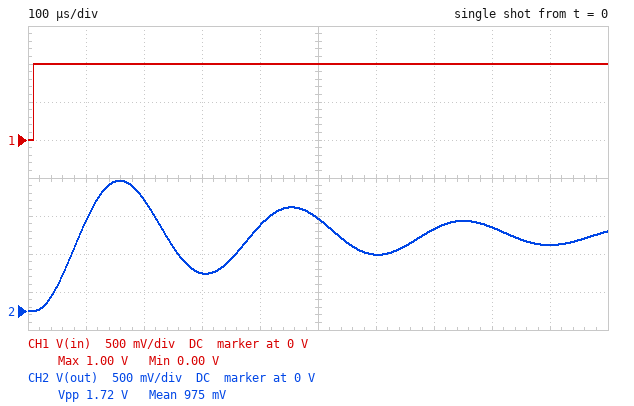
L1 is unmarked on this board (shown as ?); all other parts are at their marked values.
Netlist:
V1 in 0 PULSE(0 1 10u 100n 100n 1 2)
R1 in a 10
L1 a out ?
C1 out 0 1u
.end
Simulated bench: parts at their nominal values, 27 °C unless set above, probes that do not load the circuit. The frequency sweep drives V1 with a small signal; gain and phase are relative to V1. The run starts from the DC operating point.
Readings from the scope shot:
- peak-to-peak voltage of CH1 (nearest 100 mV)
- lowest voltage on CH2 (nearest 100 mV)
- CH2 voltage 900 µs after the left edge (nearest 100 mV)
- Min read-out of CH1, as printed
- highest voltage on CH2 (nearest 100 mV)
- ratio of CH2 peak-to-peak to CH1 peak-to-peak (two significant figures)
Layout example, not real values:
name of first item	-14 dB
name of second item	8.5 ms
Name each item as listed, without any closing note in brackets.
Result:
peak-to-peak voltage of CH1	1.0 V
lowest voltage on CH2	0 V
CH2 voltage 900 µs after the left edge	900 mV
Min read-out of CH1, as printed	0.00 V
highest voltage on CH2	1.7 V
ratio of CH2 peak-to-peak to CH1 peak-to-peak	1.7
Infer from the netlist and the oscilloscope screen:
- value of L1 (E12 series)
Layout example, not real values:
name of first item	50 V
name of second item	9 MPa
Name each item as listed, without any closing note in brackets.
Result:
value of L1	2.2 mH
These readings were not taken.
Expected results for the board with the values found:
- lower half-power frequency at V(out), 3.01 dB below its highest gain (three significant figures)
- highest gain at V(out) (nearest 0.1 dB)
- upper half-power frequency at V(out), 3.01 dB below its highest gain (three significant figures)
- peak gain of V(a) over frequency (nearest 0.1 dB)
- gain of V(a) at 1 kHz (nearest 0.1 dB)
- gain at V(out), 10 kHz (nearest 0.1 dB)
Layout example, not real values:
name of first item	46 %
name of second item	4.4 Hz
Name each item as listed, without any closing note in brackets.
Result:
lower half-power frequency at V(out), 3.01 dB below its highest gain	2.97 kHz
highest gain at V(out)	13.5 dB
upper half-power frequency at V(out), 3.01 dB below its highest gain	3.70 kHz
peak gain of V(a) over frequency	0 dB
gain of V(a) at 1 kHz	0 dB
gain at V(out), 10 kHz	-17.7 dB
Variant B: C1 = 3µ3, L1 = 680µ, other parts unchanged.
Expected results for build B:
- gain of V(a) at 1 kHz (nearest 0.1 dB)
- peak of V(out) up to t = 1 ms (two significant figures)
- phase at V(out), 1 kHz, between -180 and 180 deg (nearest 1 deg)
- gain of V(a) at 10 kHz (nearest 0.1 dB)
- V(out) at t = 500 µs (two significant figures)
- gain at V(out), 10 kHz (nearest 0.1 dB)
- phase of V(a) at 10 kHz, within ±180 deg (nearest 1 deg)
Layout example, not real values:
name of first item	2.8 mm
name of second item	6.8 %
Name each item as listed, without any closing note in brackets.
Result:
gain of V(a) at 1 kHz	-0.2 dB
peak of V(out) up to t = 1 ms	1.3 V
phase at V(out), 1 kHz, between -180 and 180 deg	-13 deg
gain of V(a) at 10 kHz	-0.3 dB
V(out) at t = 500 µs	1.0 V
gain at V(out), 10 kHz	-18.2 dB
phase of V(a) at 10 kHz, within ±180 deg	15 deg
